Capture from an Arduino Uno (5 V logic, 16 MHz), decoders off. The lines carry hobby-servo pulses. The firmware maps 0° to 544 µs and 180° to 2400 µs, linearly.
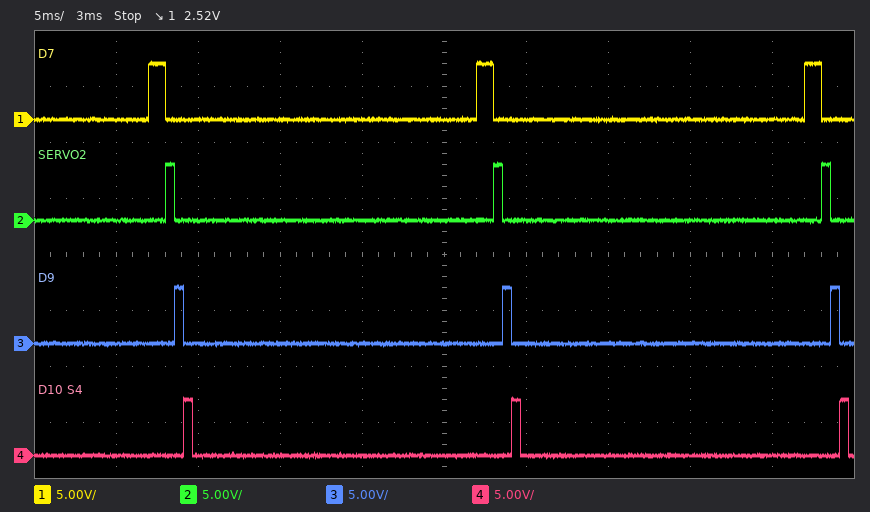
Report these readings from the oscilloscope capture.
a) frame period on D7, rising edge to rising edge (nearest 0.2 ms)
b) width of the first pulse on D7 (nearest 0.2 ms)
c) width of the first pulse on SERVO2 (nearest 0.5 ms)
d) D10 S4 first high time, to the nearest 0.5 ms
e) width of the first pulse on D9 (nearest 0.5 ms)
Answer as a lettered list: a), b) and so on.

a) 20.0 ms
b) 1.0 ms
c) 0.5 ms
d) 0.5 ms
e) 0.5 ms
